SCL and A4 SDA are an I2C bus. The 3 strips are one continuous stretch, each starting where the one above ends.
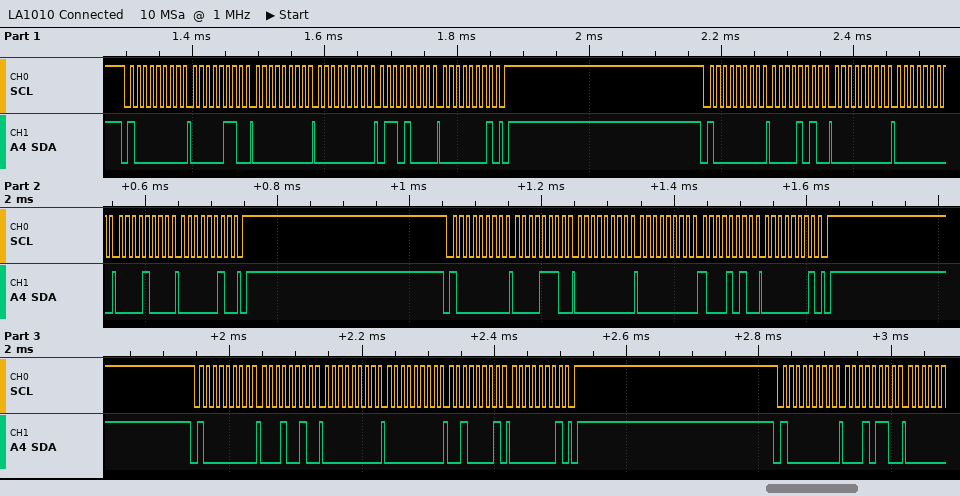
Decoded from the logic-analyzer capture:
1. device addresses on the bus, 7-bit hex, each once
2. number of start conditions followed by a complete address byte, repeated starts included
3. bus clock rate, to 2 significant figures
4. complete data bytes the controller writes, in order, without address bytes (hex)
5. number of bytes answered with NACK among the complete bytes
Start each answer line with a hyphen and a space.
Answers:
- 0x40
- 5
- 100 kHz
- 06 00 00 68 01 0A 00 00 08 02 0E 00 00 8A 01 12 00 00 21 01 16
- 0
